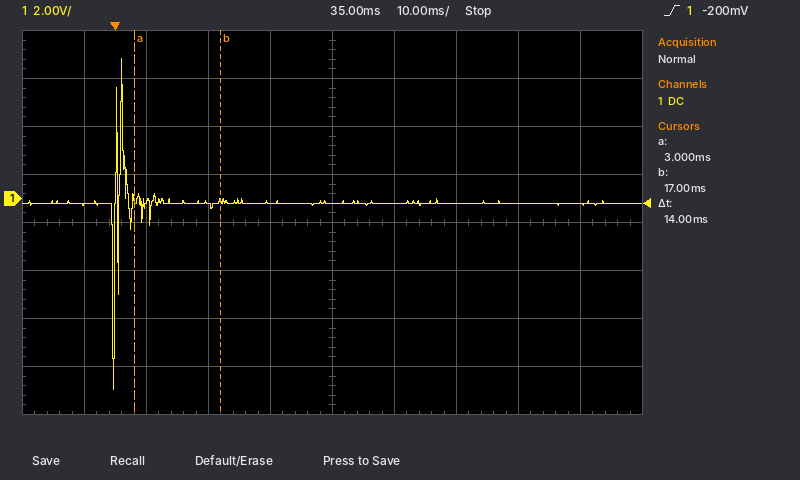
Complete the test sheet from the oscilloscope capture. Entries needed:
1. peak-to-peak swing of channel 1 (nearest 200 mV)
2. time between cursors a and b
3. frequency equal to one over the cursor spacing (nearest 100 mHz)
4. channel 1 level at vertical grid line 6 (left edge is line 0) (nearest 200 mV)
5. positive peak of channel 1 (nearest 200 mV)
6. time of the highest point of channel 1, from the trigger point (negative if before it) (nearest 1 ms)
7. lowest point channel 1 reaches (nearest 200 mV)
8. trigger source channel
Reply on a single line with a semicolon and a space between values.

13.8 V; 14 ms; 71.4 Hz; -200 mV; 5.8 V; +1 ms; -8.0 V; channel 1
